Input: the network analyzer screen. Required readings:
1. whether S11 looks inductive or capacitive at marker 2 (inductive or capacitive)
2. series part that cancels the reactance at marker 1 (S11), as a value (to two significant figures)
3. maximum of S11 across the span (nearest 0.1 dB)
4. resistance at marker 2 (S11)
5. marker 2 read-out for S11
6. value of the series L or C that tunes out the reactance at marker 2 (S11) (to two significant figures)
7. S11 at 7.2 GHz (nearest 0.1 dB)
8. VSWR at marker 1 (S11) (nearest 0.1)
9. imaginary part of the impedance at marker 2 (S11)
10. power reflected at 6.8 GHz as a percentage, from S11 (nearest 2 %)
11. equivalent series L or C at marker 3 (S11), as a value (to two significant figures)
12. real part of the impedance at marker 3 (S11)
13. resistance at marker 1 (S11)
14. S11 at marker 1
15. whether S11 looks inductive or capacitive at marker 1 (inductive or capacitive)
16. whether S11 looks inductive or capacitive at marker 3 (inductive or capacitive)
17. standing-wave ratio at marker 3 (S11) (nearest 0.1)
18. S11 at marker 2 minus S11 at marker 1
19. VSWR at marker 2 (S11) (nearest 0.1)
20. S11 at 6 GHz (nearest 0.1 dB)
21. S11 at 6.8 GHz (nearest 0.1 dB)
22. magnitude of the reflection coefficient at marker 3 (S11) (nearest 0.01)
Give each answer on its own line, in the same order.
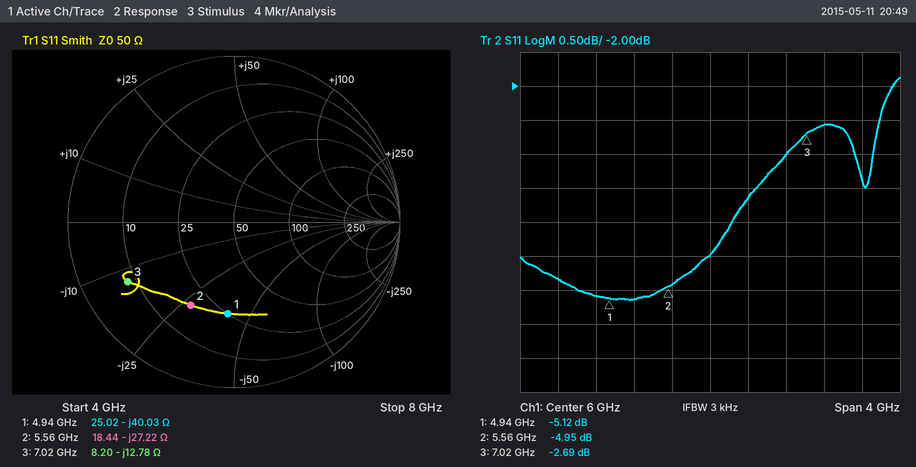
capacitive
1.3 nH
-1.9 dB
18.44 Ω
-4.95 dB
780 pH
-2.6 dB
3.5
-27.22 Ω
50 %
1.8 pF
8.20 Ω
25.02 Ω
-5.12 dB
capacitive
capacitive
6.5
0.17 dB
3.6
-4.5 dB
-3.0 dB
0.73
